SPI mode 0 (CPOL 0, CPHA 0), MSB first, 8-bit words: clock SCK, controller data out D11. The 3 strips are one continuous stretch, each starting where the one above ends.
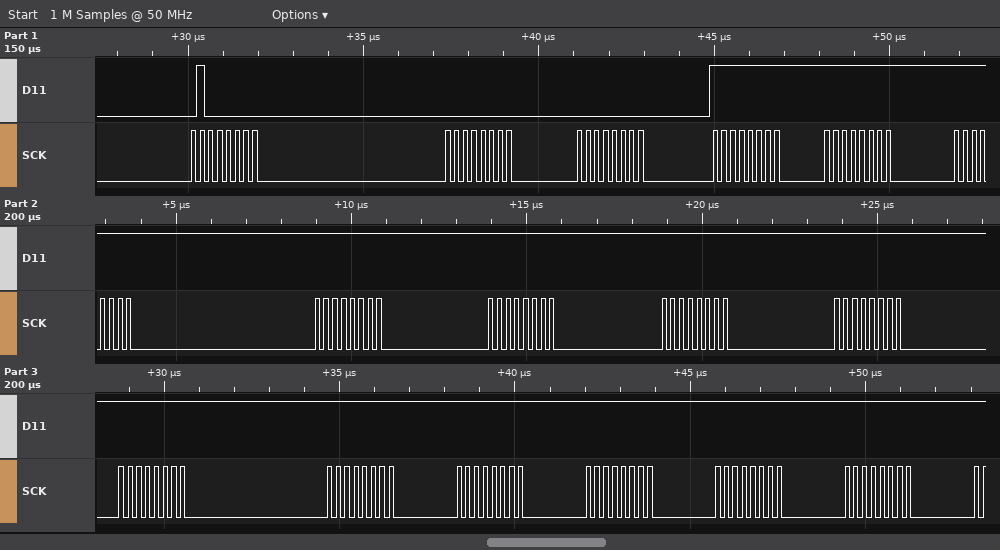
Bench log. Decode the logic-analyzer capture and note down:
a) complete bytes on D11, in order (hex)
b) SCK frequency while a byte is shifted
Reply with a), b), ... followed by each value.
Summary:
a) 0x40 0x00 0x00 0xFF 0xFF 0xFF 0xFF 0xFF 0xFF 0xFF 0xFF 0xFF 0xFF 0xFF 0xFF 0xFF
b) 4 MHz
